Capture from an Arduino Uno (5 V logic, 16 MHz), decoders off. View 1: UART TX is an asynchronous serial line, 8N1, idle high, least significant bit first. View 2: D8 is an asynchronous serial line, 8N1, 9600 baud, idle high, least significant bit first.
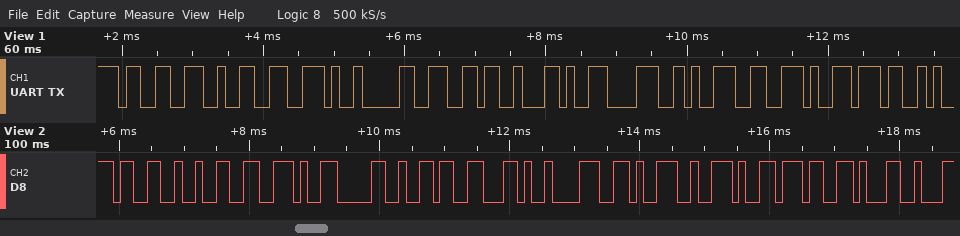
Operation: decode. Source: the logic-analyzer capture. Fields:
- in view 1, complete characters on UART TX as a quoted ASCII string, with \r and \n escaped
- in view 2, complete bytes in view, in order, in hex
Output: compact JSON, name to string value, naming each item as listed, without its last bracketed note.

{"in view 1, complete characters on UART TX as a quoted ASCII string, with \\r and \\n escaped": "\"32.06,89.7\"", "in view 2, complete bytes in view, in order, in hex": "0x33 0x32 0x2E 0x30 0x36 0x2C 0x38 0x39 0x2E 0x37 0x31"}
